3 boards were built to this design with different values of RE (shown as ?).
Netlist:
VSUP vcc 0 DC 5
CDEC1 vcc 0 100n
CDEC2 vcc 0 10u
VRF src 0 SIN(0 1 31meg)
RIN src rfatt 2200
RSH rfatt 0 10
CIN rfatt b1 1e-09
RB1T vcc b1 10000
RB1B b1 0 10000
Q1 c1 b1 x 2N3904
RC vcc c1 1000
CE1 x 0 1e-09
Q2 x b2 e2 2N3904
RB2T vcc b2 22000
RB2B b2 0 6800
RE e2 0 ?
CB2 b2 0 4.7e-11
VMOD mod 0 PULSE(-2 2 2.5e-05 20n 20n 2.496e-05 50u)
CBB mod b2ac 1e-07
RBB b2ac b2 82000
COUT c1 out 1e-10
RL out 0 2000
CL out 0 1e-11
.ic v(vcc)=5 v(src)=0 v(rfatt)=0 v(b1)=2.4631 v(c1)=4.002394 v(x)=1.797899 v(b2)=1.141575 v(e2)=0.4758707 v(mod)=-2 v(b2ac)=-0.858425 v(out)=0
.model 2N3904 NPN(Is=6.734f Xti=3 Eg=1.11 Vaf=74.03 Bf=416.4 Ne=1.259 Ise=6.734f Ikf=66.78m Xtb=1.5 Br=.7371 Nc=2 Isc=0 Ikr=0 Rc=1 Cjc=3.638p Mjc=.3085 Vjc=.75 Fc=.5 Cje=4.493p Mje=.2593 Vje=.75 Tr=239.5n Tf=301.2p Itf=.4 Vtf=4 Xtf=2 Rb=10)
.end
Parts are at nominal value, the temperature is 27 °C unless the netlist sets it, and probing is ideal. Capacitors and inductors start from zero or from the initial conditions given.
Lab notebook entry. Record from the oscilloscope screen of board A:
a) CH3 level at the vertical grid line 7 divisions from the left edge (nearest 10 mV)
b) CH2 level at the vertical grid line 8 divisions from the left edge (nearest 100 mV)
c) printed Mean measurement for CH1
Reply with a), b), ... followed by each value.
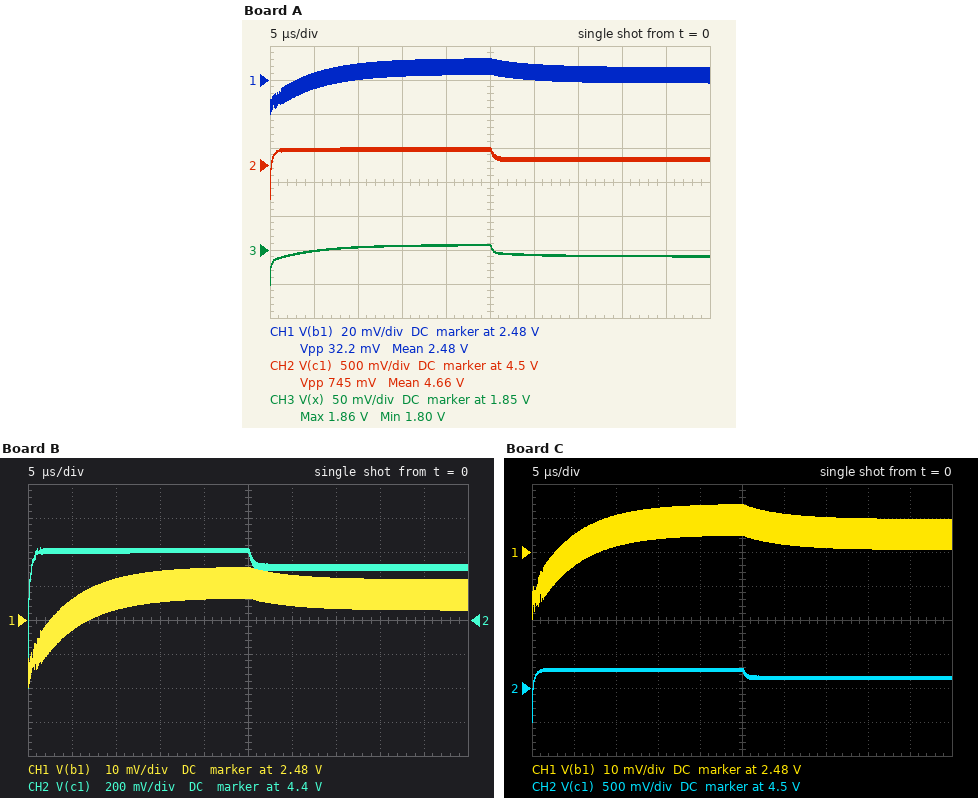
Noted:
a) 1.84 V
b) 4.6 V
c) 2.48 V
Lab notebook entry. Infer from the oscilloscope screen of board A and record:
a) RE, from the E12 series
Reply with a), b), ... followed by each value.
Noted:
a) 1.5 kΩ
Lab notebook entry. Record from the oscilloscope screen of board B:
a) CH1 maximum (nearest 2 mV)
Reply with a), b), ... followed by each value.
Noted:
a) 2.496 V
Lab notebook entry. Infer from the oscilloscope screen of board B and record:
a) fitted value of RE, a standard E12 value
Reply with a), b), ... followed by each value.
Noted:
a) 2.2 kΩ
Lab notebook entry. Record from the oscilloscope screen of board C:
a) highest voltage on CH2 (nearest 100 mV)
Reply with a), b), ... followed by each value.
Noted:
a) 4.8 V
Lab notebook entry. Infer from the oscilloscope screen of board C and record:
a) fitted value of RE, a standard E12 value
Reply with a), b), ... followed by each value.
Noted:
a) 1.8 kΩ
